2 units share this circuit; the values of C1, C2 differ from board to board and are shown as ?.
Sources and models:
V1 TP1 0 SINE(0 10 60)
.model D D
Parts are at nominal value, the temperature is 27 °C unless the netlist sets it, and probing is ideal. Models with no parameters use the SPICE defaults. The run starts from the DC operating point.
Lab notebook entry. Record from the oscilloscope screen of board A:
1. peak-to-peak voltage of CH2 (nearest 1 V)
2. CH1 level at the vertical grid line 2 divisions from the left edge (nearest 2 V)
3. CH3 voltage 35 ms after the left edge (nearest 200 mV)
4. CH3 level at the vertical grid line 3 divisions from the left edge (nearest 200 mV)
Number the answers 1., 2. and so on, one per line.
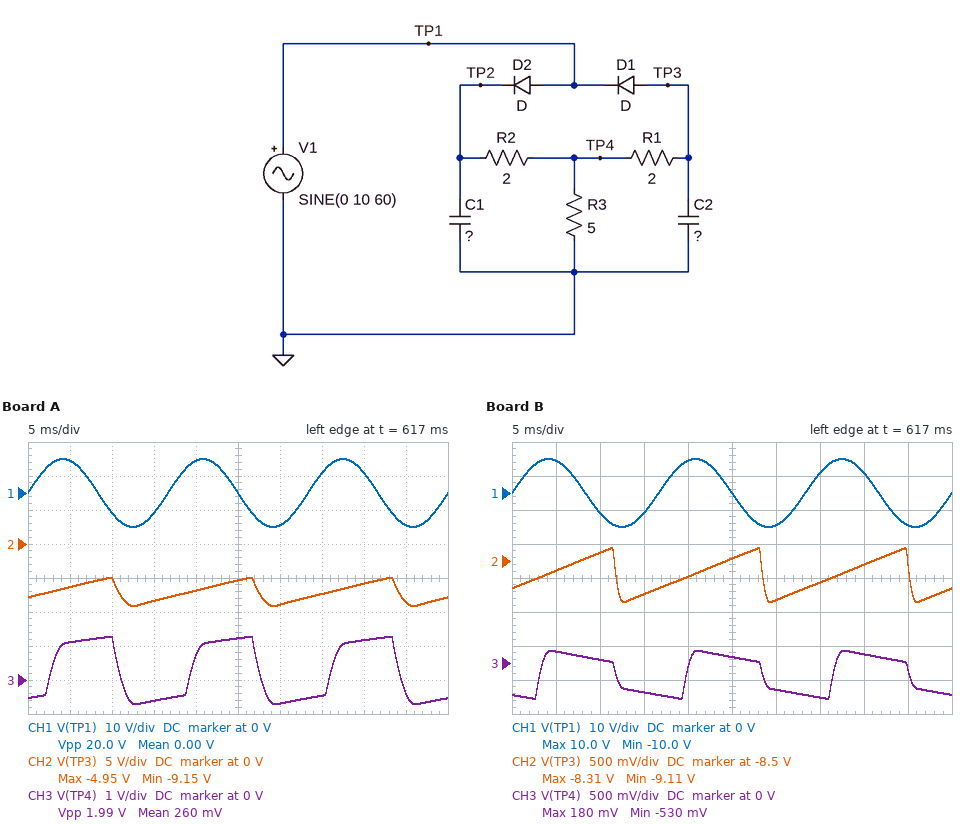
1. 4 V
2. -6 V
3. -400 mV
4. -600 mV
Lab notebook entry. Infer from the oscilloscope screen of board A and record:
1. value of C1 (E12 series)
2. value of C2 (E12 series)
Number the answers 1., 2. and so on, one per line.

1. 18 mF
2. 12 mF
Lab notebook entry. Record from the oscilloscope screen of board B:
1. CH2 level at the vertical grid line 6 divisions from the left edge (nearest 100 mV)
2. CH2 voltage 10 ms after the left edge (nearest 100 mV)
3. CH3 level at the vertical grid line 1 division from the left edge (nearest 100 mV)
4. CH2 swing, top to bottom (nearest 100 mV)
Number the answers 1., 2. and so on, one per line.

1. -9.1 V
2. -8.4 V
3. 200 mV
4. 800 mV
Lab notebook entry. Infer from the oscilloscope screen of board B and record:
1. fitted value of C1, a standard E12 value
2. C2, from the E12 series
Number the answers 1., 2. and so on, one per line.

1. 39 mF
2. 82 mF
